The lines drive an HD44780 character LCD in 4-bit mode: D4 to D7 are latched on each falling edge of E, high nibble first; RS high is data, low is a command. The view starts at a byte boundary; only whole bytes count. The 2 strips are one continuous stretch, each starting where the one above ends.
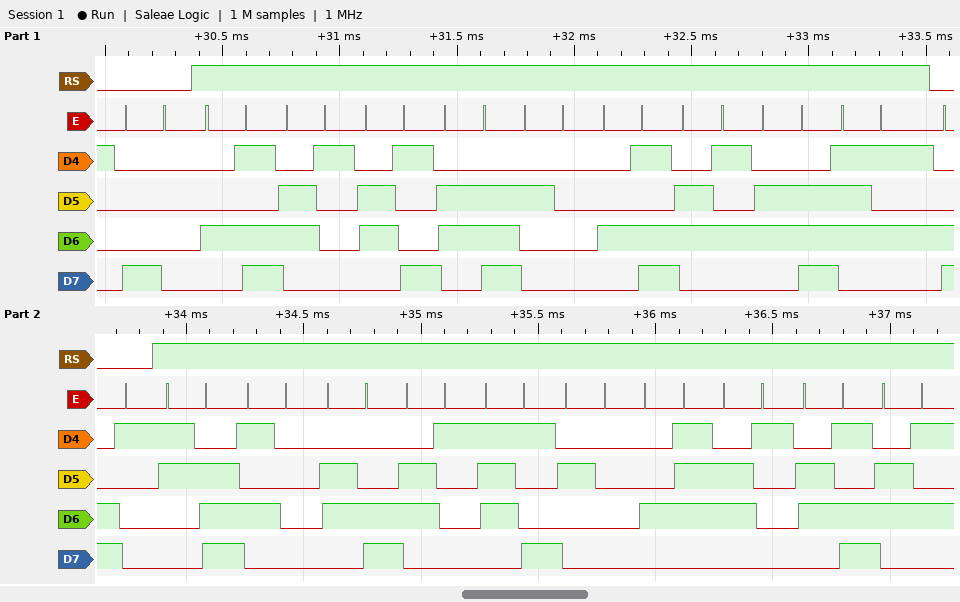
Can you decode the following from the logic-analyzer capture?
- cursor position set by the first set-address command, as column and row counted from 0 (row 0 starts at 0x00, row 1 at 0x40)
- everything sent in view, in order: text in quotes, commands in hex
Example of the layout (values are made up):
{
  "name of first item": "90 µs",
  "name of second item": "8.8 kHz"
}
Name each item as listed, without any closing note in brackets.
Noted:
{
  "cursor position set by the first set-address command, as column and row counted from 0": "column 0, row 0",
  "everything sent in view, in order: text in quotes, commands in hex": "0x80 \"Main Menu\" 0xC1 \">Play Game\""
}
